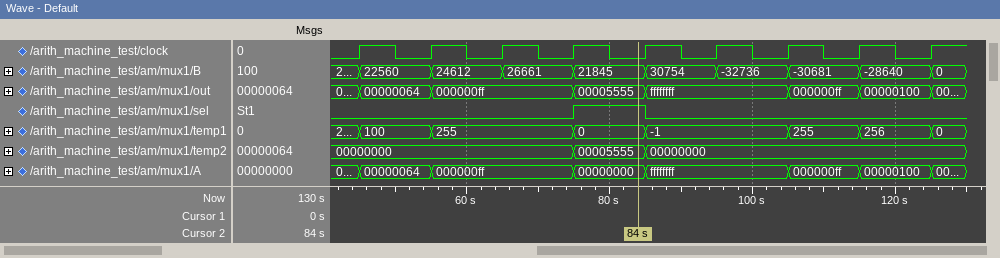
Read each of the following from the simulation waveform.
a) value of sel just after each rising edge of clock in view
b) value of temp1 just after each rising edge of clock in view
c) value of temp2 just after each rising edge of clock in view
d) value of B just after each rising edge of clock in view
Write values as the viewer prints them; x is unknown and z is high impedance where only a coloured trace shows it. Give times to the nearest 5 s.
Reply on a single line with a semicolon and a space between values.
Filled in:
0 0 0 1 0 0 0 0 0; 100, 255, 255, 0, -1, -1, 255, 256, 0; 00000000, 00000000, 00000000, 00005555, 00000000, 00000000, 00000000, 00000000, 00000000; 22560, 24612, 26661, 21845, 30754, -32736, -30681, -28640, 0
